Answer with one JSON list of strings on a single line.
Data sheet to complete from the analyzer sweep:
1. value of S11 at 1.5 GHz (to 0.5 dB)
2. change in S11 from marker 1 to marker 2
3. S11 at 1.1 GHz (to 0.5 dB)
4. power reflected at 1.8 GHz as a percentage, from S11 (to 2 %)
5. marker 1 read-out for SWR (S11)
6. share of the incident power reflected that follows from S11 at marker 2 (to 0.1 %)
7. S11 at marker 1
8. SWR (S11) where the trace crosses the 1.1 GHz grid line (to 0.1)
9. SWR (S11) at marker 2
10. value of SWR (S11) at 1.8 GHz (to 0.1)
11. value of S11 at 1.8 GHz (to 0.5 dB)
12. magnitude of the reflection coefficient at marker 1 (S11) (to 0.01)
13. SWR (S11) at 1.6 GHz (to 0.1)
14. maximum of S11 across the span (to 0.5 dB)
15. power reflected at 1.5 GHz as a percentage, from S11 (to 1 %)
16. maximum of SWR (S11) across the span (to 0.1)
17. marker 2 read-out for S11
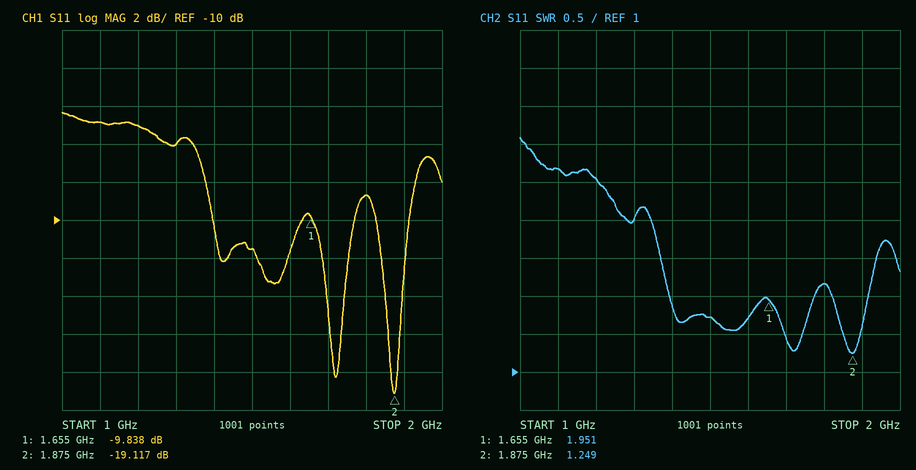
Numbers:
["-11.5 dB", "-9.279 dB", "-5.0 dB", "14 %", "1.951", "1.2 %", "-9.838 dB", "3.7", "1.249", "2.2", "-8.5 dB", "0.32", "1.7", "-4.5 dB", "7 %", "4.1", "-19.117 dB"]
